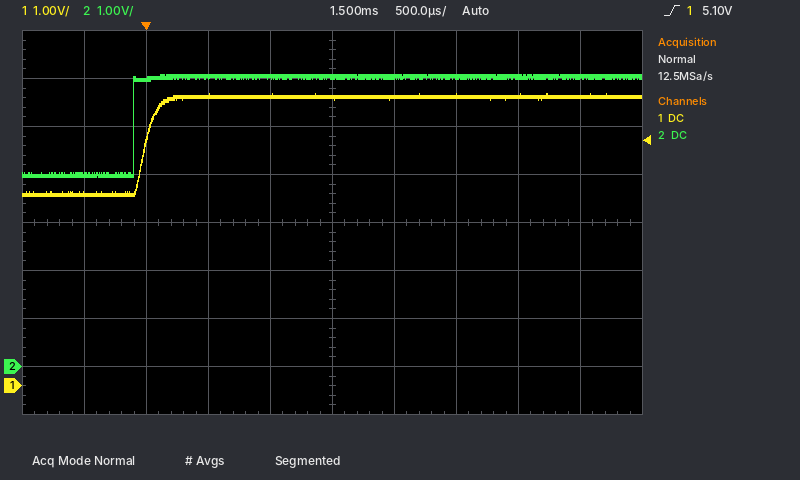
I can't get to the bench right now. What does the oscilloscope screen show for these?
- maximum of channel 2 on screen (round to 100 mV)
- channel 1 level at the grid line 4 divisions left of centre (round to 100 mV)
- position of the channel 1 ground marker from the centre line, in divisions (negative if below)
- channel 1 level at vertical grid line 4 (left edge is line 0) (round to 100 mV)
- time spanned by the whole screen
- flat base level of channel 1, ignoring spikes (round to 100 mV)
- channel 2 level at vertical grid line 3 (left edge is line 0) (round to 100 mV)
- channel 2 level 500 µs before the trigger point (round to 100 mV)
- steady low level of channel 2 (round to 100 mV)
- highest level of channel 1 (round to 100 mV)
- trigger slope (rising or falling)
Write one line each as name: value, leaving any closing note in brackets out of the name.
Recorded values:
maximum of channel 2 on screen: 6.1 V
channel 1 level at the grid line 4 divisions left of centre: 4.0 V
position of the channel 1 ground marker from the centre line, in divisions: -3.4 div
channel 1 level at vertical grid line 4 (left edge is line 0): 6.0 V
time spanned by the whole screen: 5 ms
flat base level of channel 1, ignoring spikes: 4.0 V
channel 2 level at vertical grid line 3 (left edge is line 0): 6.0 V
channel 2 level 500 µs before the trigger point: 4.0 V
steady low level of channel 2: 4.0 V
highest level of channel 1: 6.1 V
trigger slope: rising
